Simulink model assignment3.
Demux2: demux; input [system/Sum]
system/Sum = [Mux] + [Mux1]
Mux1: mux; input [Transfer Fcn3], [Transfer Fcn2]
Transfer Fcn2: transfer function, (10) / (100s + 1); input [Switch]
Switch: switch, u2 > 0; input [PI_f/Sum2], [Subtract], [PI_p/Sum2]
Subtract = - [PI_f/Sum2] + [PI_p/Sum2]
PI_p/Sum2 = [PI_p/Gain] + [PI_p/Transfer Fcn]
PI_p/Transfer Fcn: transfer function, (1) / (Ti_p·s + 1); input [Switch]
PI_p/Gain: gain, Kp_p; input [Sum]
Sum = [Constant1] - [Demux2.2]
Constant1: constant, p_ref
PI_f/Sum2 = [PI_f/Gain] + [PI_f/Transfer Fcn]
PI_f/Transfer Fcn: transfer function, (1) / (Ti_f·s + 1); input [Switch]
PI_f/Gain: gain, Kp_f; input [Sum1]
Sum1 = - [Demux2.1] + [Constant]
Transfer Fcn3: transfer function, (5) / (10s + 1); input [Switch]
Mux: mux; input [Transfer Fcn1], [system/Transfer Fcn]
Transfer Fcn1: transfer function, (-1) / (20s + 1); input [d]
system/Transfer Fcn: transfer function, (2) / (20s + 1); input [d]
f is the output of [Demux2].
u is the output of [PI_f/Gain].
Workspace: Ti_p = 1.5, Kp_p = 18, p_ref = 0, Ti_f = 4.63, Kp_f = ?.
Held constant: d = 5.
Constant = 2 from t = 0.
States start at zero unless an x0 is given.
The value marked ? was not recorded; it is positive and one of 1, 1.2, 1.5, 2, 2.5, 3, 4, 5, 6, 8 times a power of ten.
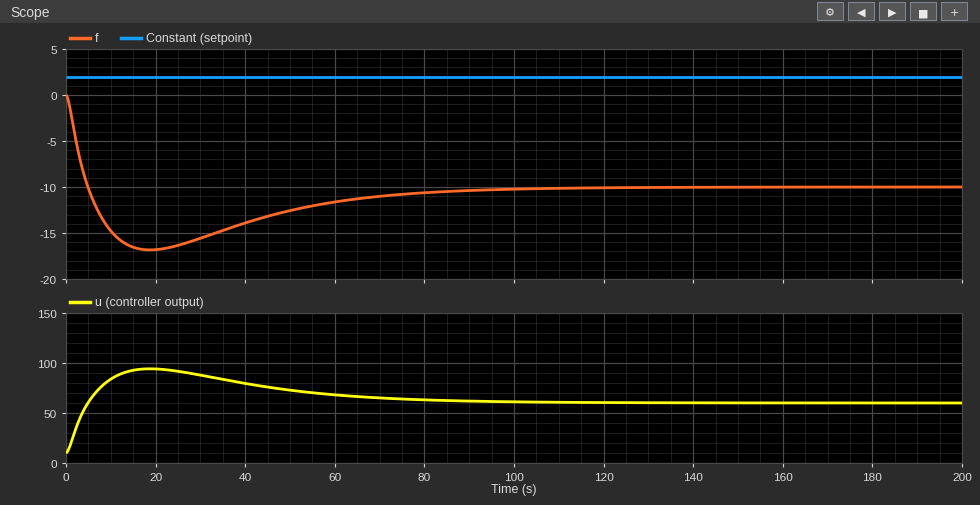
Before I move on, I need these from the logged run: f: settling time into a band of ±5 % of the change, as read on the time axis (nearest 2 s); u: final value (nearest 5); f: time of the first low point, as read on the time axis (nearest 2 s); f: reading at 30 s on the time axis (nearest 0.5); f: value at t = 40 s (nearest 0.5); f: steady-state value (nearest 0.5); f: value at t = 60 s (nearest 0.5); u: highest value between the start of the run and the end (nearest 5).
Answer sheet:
84 s
60
18 s
-15.5
-14.0
-10.0
-11.5
95
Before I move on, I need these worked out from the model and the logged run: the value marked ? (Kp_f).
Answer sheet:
5
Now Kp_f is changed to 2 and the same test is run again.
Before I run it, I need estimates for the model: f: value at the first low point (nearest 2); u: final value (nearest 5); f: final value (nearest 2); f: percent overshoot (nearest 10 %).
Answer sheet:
-16
25
-10
70 %
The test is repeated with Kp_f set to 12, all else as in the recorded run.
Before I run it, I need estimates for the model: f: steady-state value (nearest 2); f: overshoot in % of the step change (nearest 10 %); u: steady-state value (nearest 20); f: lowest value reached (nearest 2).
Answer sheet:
-10
70 %
140
-16
